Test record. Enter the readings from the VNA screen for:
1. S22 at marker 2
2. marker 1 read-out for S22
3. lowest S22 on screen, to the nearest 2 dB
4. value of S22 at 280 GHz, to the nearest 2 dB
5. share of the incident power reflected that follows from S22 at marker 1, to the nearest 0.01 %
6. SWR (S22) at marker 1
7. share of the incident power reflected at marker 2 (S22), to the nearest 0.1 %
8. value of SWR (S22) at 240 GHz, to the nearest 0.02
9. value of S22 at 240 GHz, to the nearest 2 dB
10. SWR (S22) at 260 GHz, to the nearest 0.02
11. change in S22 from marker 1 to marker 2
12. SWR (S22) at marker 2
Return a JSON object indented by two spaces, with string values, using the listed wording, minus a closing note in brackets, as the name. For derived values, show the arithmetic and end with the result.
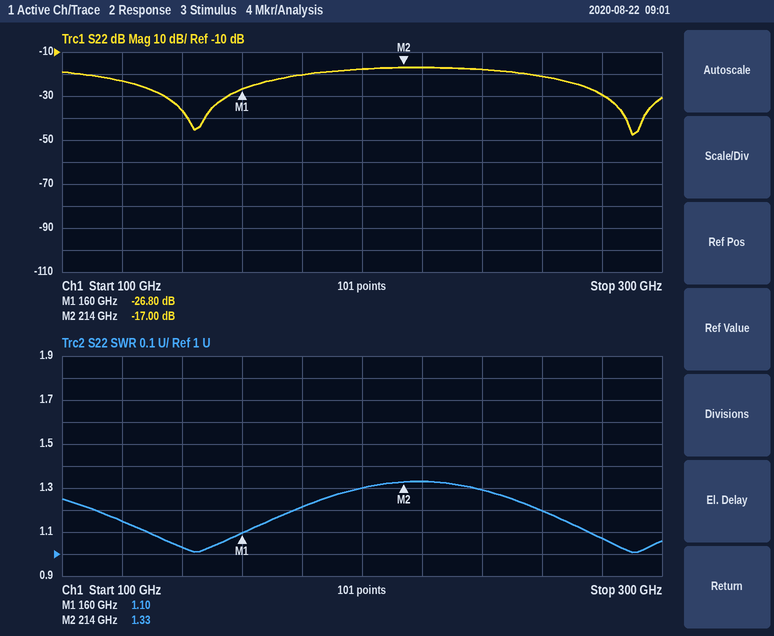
{
  "S22 at marker 2": "-17.00 dB",
  "marker 1 read-out for S22": "-26.80 dB",
  "lowest S22 on screen, to the nearest 2 dB": "-48 dB",
  "value of S22 at 280 GHz, to the nearest 2 dB": "-30 dB",
  "share of the incident power reflected that follows from S22 at marker 1, to the nearest 0.01 %": "10^(-26.8/10) ≈ 0.21 %",
  "SWR (S22) at marker 1": "1.10",
  "share of the incident power reflected at marker 2 (S22), to the nearest 0.1 %": "10^(-17/10) ≈ 2.0 %",
  "value of SWR (S22) at 240 GHz, to the nearest 0.02": "1.30",
  "value of S22 at 240 GHz, to the nearest 2 dB": "-18 dB",
  "SWR (S22) at 260 GHz, to the nearest 0.02": "1.20",
  "change in S22 from marker 1 to marker 2": "-17 − (-26.8) = 9.80 dB",
  "SWR (S22) at marker 2": "1.33"
}
